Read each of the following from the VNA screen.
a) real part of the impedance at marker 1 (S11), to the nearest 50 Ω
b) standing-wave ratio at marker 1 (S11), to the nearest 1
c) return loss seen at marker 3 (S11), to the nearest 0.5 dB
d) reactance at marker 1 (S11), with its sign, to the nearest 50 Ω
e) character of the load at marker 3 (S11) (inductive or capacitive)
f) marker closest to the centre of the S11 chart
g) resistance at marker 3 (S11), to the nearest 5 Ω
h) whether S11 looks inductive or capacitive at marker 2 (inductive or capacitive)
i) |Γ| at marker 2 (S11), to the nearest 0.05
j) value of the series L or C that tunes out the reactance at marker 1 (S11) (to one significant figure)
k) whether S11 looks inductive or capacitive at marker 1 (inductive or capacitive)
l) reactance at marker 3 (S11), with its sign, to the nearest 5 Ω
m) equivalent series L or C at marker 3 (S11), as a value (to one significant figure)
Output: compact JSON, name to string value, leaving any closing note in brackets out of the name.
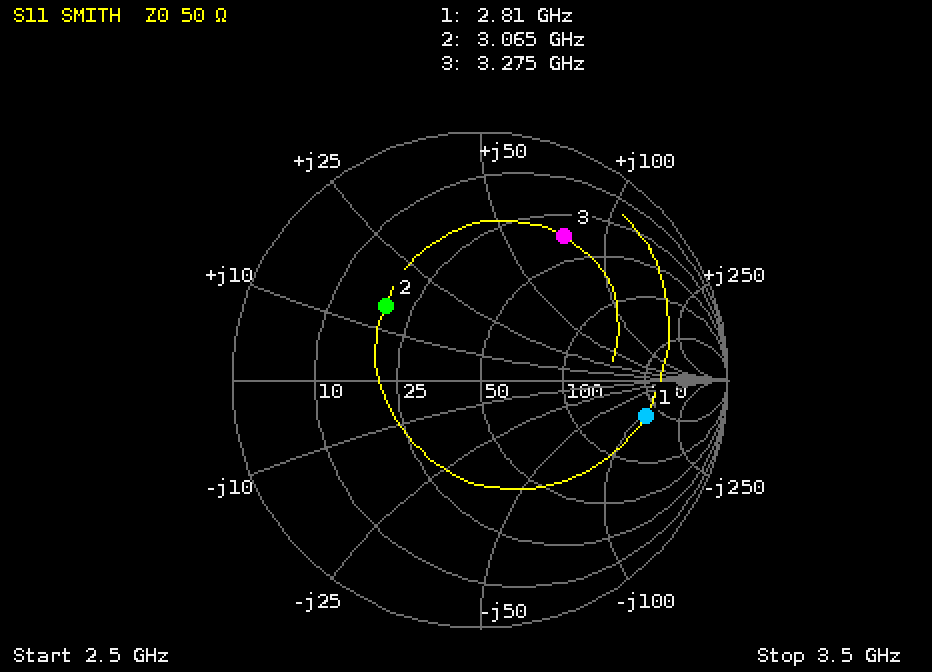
{"real part of the impedance at marker 1 (S11), to the nearest 50 Ω": "200 Ω", "standing-wave ratio at marker 1 (S11), to the nearest 1": "5", "return loss seen at marker 3 (S11), to the nearest 0.5 dB": "3.5 dB", "reactance at marker 1 (S11), with its sign, to the nearest 50 Ω": "-100 Ω", "character of the load at marker 3 (S11)": "inductive", "marker closest to the centre of the S11 chart": "marker 2", "resistance at marker 3 (S11), to the nearest 5 Ω": "35 Ω", "whether S11 looks inductive or capacitive at marker 2": "inductive", "|Γ| at marker 2 (S11), to the nearest 0.05": "0.50", "value of the series L or C that tunes out the reactance at marker 1 (S11)": "6 nH", "whether S11 looks inductive or capacitive at marker 1": "capacitive", "reactance at marker 3 (S11), with its sign, to the nearest 5 Ω": "+75 Ω", "equivalent series L or C at marker 3 (S11), as a value": "4 nH"}
